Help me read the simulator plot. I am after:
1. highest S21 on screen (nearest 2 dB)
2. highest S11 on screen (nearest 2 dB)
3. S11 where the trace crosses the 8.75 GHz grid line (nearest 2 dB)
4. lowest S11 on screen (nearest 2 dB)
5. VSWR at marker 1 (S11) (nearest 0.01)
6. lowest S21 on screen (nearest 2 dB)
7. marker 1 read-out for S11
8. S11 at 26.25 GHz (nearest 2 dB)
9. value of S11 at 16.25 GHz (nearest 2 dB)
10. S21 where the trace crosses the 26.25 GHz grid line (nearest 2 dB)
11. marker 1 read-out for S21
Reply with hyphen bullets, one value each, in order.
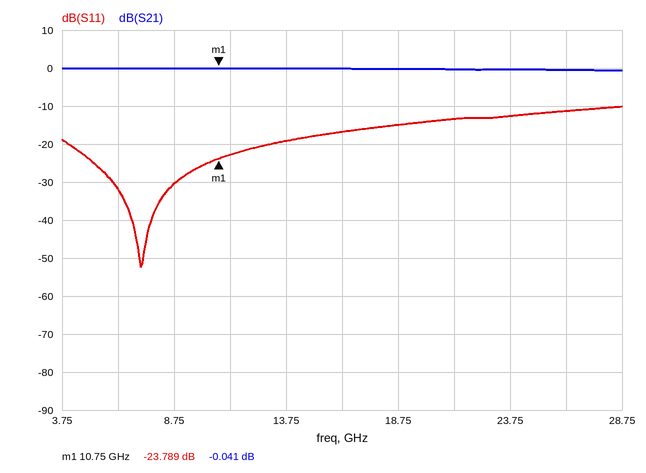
- 0 dB
- -10 dB
- -30 dB
- -52 dB
- 1.14
- 0 dB
- -23.789 dB
- -12 dB
- -16 dB
- 0 dB
- -0.041 dB
